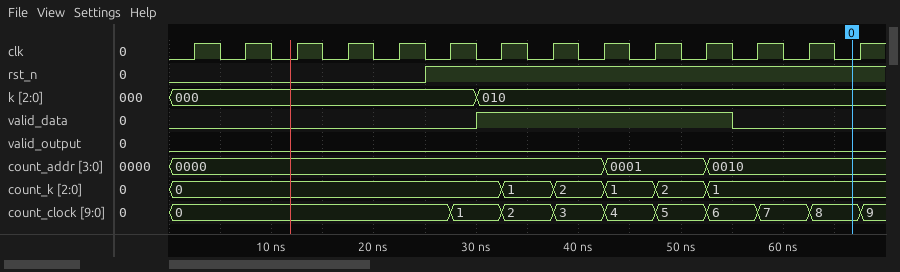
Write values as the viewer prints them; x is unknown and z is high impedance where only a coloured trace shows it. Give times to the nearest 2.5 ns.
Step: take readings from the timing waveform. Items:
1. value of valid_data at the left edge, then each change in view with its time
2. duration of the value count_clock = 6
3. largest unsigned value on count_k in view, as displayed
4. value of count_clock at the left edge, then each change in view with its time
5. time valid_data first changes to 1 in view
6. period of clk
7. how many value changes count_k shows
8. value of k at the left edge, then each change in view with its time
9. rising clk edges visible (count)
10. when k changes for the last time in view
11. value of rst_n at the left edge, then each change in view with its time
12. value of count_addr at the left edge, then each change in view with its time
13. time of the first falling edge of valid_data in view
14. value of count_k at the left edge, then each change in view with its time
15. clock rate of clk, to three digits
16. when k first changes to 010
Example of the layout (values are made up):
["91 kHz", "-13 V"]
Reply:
["0, 1 at 30 ns, 0 at 55 ns", "5 ns", "2", "0, 1 at 27.5 ns, 2 at 32.5 ns, 3 at 37.5 ns, 4 at 42.5 ns, 5 at 47.5 ns, 6 at 52.5 ns, 7 at 57.5 ns, 8 at 62.5 ns, 9 at 67.5 ns", "30 ns", "5 ns", "5", "000, 010 at 30 ns", "14", "30 ns", "0, 1 at 25 ns", "0000, 0001 at 42.5 ns, 0010 at 52.5 ns", "55 ns", "0, 1 at 32.5 ns, 2 at 37.5 ns, 1 at 42.5 ns, 2 at 47.5 ns, 1 at 52.5 ns", "200 MHz", "30 ns"]
